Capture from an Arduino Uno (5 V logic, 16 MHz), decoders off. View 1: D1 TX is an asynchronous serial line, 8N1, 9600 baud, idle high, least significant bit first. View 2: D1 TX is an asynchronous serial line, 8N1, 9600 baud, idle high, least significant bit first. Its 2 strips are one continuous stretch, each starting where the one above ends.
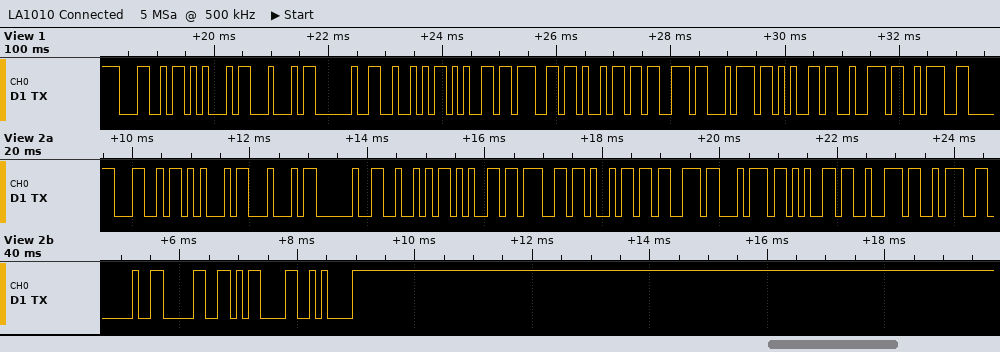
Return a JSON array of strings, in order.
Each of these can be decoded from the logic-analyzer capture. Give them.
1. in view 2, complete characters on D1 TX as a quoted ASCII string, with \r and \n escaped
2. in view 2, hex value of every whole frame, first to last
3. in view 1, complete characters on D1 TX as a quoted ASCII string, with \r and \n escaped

["\"LED Register: 0\\r\\n\"", "0x4C 0x45 0x44 0x20 0x52 0x65 0x67 0x69 0x73 0x74 0x65 0x72 0x3A 0x20 0x30 0x0D 0x0A", "\"LED Register:\""]
